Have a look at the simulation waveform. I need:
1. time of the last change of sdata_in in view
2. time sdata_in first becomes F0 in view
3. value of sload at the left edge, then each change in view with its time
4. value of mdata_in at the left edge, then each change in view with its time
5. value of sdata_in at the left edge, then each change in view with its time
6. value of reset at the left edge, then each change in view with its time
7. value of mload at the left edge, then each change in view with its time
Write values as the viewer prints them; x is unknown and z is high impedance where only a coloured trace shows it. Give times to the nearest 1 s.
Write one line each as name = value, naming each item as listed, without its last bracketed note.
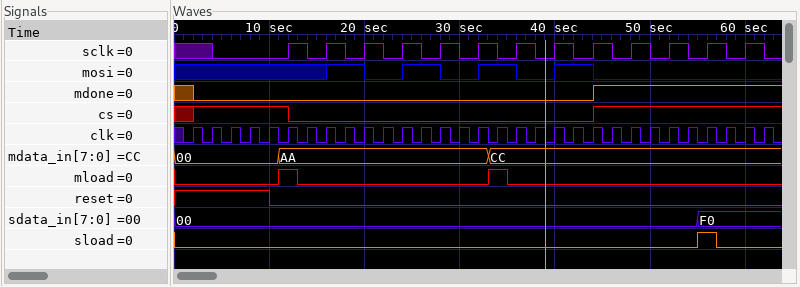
time of the last change of sdata_in in view = 55 s
time sdata_in first becomes F0 in view = 55 s
value of sload at the left edge, then each change in view with its time = 0, 1 at 55 s, 0 at 57 s
value of mdata_in at the left edge, then each change in view with its time = 00, AA at 11 s, CC at 33 s
value of sdata_in at the left edge, then each change in view with its time = 00, F0 at 55 s
value of reset at the left edge, then each change in view with its time = 1, 0 at 10 s
value of mload at the left edge, then each change in view with its time = 0, 1 at 11 s, 0 at 13 s, 1 at 33 s, 0 at 35 s
